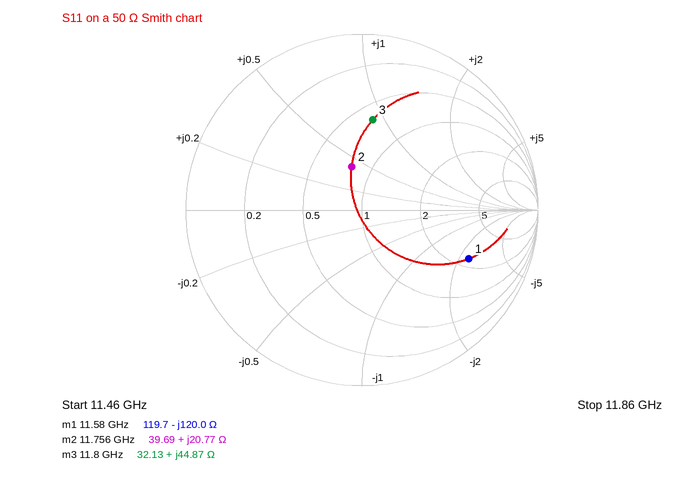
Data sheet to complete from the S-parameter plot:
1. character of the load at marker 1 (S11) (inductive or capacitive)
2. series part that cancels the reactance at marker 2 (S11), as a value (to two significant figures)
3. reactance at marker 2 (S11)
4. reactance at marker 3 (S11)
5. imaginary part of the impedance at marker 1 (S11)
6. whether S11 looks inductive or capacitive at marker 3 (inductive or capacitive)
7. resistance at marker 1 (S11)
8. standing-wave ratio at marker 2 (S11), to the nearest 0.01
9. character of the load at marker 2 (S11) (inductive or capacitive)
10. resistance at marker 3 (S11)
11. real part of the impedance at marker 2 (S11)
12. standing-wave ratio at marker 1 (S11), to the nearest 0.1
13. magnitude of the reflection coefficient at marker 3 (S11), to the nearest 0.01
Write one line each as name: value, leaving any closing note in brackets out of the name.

character of the load at marker 1 (S11): capacitive
series part that cancels the reactance at marker 2 (S11), as a value: 650 fF
reactance at marker 2: +20.77 Ω
reactance at marker 3: +44.87 Ω
imaginary part of the impedance at marker 1: -120.0 Ω
whether S11 looks inductive or capacitive at marker 3: inductive
resistance at marker 1: 119.7 Ω
standing-wave ratio at marker 2 (S11), to the nearest 0.01: 1.67
character of the load at marker 2 (S11): inductive
resistance at marker 3: 32.13 Ω
real part of the impedance at marker 2: 39.69 Ω
standing-wave ratio at marker 1 (S11), to the nearest 0.1: 5.0
magnitude of the reflection coefficient at marker 3 (S11), to the nearest 0.01: 0.52
